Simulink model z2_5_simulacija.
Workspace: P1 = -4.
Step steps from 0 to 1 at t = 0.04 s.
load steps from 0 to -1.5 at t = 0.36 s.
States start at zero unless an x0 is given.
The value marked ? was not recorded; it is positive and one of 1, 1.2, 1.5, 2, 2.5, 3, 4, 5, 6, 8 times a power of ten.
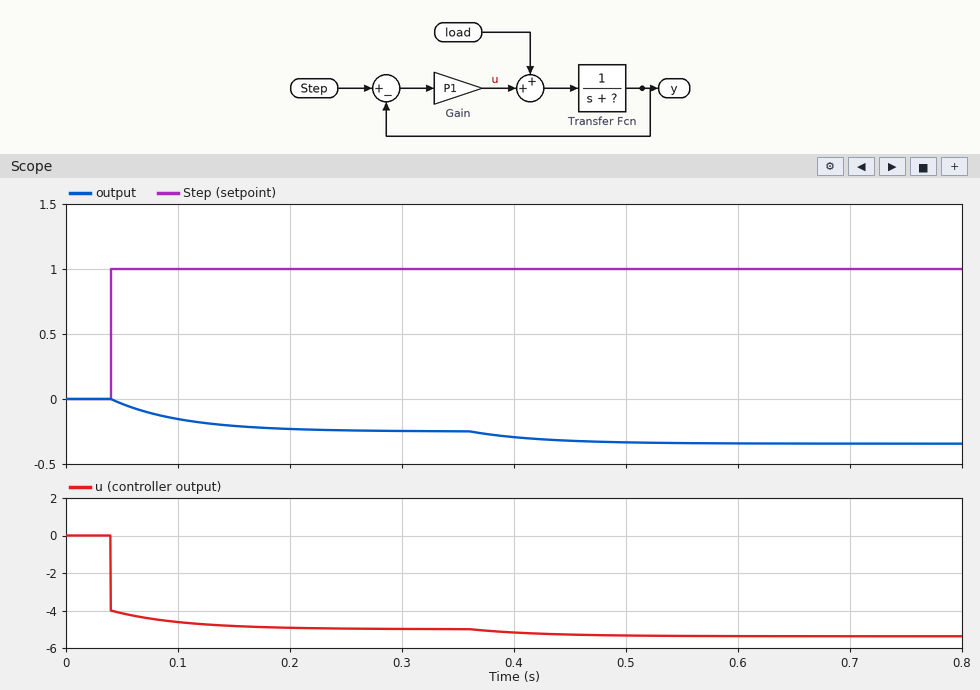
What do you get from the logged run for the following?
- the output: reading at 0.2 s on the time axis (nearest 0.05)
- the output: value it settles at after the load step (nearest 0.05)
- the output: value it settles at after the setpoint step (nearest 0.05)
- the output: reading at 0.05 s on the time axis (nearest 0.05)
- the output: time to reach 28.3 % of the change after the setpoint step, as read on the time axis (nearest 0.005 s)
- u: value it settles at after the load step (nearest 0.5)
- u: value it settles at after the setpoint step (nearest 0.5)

-0.25
-0.35
-0.25
-0.05
0.060 s
-5.5
-5.0
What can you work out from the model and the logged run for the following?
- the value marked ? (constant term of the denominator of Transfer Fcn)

20
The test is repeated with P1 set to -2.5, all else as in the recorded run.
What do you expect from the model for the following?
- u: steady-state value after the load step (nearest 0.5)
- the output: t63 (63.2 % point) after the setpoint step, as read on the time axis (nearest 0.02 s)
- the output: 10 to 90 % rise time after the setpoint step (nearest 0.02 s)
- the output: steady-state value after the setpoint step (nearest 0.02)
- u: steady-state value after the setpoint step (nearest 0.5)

-3.0
0.10 s
0.12 s
-0.14
-3.0
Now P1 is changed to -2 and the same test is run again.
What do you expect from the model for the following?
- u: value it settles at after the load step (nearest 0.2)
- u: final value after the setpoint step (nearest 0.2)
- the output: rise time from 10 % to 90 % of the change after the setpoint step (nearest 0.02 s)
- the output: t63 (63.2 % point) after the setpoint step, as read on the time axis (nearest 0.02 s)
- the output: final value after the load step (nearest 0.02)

-2.4
-2.2
0.12 s
0.10 s
-0.20
